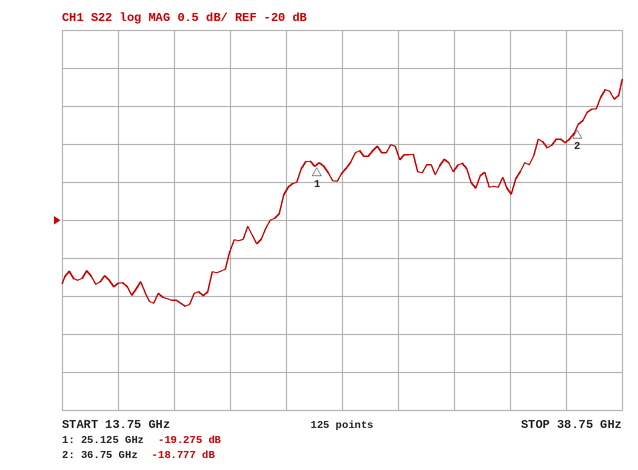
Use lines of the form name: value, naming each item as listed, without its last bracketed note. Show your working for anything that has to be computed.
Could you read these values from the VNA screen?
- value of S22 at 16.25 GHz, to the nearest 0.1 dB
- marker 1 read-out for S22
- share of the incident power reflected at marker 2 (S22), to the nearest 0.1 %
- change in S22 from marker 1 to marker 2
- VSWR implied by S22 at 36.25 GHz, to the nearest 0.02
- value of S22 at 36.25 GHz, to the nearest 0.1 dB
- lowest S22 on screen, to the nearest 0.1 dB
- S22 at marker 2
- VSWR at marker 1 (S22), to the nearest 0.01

value of S22 at 16.25 GHz, to the nearest 0.1 dB: -20.8 dB
marker 1 read-out for S22: -19.275 dB
share of the incident power reflected at marker 2 (S22), to the nearest 0.1 %: 10^(-18.777/10) ≈ 1.3 %
change in S22 from marker 1 to marker 2: -18.777 − (-19.275) = 0.498 dB
VSWR implied by S22 at 36.25 GHz, to the nearest 0.02: |Γ| = 10^(-19/20) = 0.1122; VSWR = (1 + 0.1122)/(1 − 0.1122) ≈ 1.25, so 1.26 to the nearest 0.02
value of S22 at 36.25 GHz, to the nearest 0.1 dB: -19.0 dB
lowest S22 on screen, to the nearest 0.1 dB: -21.1 dB
S22 at marker 2: -18.777 dB
VSWR at marker 1 (S22), to the nearest 0.01: (1 + 0.1087)/(1 − 0.1087) ≈ 1.24
